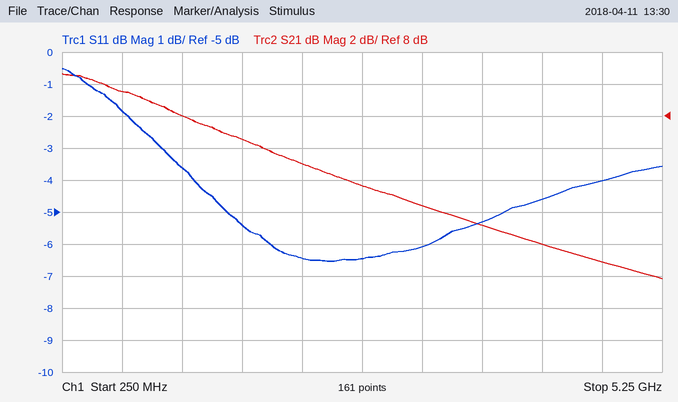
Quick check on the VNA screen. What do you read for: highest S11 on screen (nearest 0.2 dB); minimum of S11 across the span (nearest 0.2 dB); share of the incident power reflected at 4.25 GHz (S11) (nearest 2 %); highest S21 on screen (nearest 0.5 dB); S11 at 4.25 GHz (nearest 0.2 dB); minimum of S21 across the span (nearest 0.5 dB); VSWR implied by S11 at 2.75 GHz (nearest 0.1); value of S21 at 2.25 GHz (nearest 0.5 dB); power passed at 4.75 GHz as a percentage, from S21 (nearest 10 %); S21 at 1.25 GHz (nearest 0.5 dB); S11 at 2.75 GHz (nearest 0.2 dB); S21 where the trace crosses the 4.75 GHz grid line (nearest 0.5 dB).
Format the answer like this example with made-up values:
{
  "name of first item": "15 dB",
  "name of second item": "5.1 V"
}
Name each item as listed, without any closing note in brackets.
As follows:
{
  "highest S11 on screen": "-0.6 dB",
  "minimum of S11 across the span": "-6.6 dB",
  "share of the incident power reflected at 4.25 GHz (S11)": "34 %",
  "highest S21 on screen": "10.5 dB",
  "S11 at 4.25 GHz": "-4.6 dB",
  "minimum of S21 across the span": "-2.0 dB",
  "VSWR implied by S11 at 2.75 GHz": "2.8",
  "value of S21 at 2.25 GHz": "5.0 dB",
  "power passed at 4.75 GHz as a percentage, from S21": "80 %",
  "S21 at 1.25 GHz": "8.0 dB",
  "S11 at 2.75 GHz": "-6.4 dB",
  "S21 where the trace crosses the 4.75 GHz grid line": "-1.0 dB"
}
